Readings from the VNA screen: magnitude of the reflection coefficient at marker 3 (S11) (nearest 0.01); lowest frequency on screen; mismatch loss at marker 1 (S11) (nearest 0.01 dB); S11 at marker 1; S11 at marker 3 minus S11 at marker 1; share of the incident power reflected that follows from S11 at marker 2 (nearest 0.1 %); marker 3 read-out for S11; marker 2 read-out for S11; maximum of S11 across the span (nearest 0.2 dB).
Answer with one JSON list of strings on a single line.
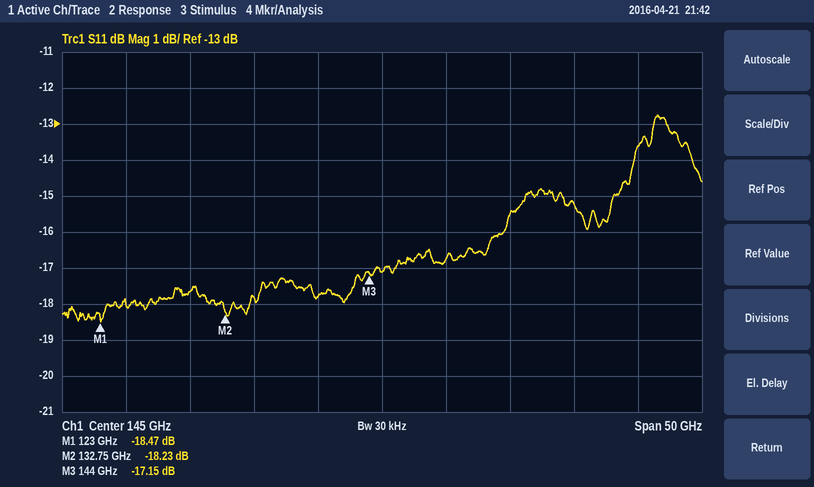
["0.14", "120 GHz", "0.06 dB", "-18.47 dB", "1.32 dB", "1.5 %", "-17.15 dB", "-18.23 dB", "-12.8 dB"]
